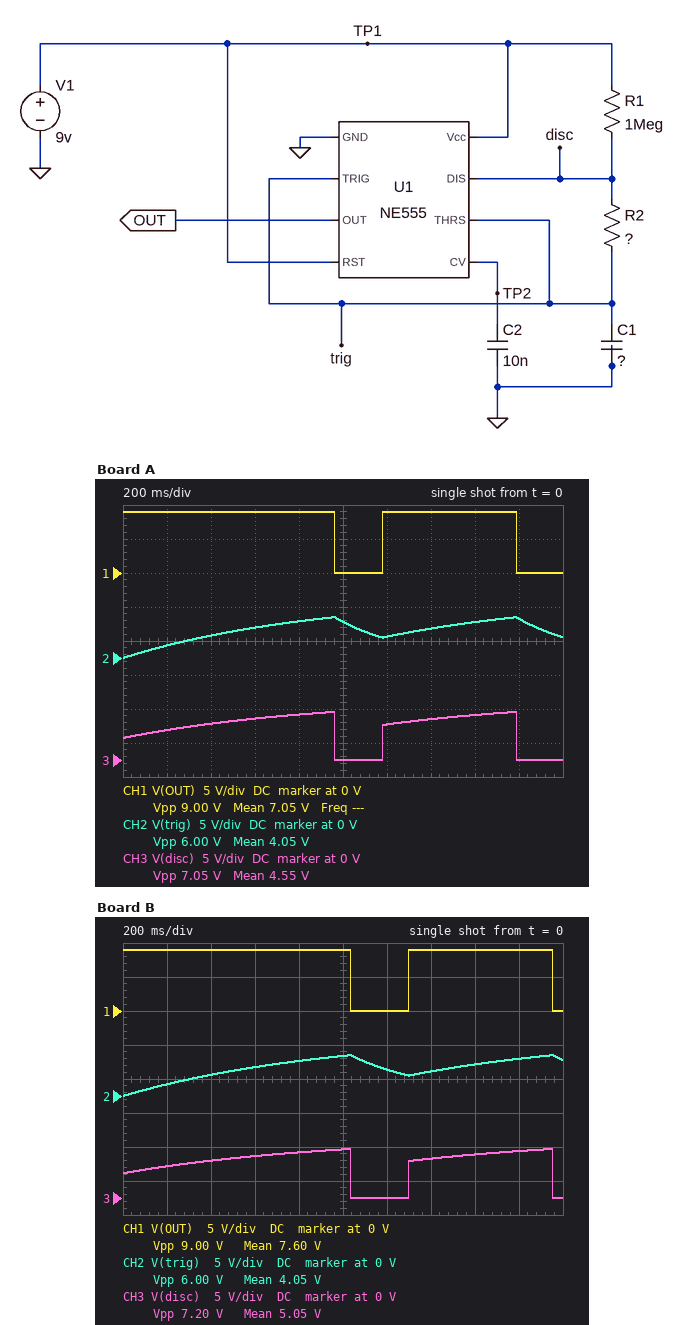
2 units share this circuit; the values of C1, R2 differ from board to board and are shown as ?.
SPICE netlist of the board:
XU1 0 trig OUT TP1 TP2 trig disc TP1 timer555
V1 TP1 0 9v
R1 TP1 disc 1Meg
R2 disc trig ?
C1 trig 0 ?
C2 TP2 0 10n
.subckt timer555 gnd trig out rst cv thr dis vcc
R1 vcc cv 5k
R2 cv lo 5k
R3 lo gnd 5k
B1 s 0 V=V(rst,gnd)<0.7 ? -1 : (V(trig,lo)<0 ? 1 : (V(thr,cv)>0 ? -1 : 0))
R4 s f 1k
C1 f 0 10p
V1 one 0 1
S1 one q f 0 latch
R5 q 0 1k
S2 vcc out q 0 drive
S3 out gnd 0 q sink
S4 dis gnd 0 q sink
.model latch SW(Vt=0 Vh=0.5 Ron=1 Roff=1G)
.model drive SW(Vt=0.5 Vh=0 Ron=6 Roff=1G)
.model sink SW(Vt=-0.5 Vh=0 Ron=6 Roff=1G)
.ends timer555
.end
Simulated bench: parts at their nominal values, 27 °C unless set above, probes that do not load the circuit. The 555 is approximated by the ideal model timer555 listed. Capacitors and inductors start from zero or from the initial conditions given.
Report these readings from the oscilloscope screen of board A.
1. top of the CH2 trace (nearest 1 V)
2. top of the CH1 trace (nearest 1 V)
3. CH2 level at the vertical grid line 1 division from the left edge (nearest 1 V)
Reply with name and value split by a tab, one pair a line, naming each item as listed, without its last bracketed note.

top of the CH2 trace	6 V
top of the CH1 trace	9 V
CH2 level at the vertical grid line 1 division from the left edge	2 V
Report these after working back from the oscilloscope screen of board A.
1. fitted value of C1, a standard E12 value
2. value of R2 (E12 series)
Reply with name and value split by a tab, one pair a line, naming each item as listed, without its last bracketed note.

fitted value of C1, a standard E12 value	560 nF
value of R2	560 kΩ
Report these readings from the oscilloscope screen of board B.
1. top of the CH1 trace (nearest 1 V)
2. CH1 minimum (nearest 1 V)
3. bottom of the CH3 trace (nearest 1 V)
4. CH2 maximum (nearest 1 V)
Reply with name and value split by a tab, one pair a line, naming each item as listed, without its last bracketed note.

top of the CH1 trace	9 V
CH1 minimum	0 V
bottom of the CH3 trace	0 V
CH2 maximum	6 V
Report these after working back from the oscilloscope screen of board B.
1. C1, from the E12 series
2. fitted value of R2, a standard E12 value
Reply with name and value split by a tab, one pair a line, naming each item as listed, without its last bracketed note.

C1, from the E12 series	560 nF
fitted value of R2, a standard E12 value	680 kΩ
